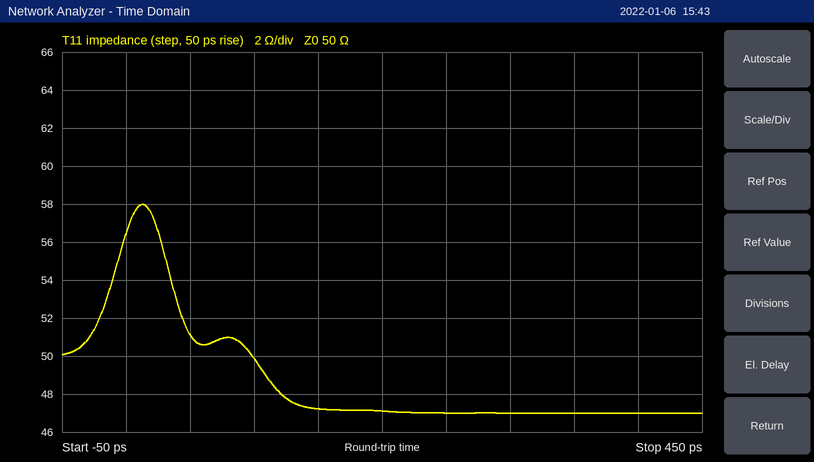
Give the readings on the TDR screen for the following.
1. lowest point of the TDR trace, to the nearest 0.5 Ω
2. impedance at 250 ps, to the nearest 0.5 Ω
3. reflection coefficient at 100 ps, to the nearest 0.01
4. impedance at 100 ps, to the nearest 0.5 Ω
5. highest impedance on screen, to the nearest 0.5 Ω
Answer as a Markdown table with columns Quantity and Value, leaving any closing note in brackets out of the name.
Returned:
| Quantity | Value |
|---|---|
| lowest point of the TDR trace, to the nearest 0.5 Ω | 47.0 Ω |
| impedance at 250 ps, to the nearest 0.5 Ω | 47.0 Ω |
| reflection coefficient at 100 ps, to the nearest 0.01 | 0.00 |
| impedance at 100 ps, to the nearest 0.5 Ω | 50.0 Ω |
| highest impedance on screen, to the nearest 0.5 Ω | 58.0 Ω |
